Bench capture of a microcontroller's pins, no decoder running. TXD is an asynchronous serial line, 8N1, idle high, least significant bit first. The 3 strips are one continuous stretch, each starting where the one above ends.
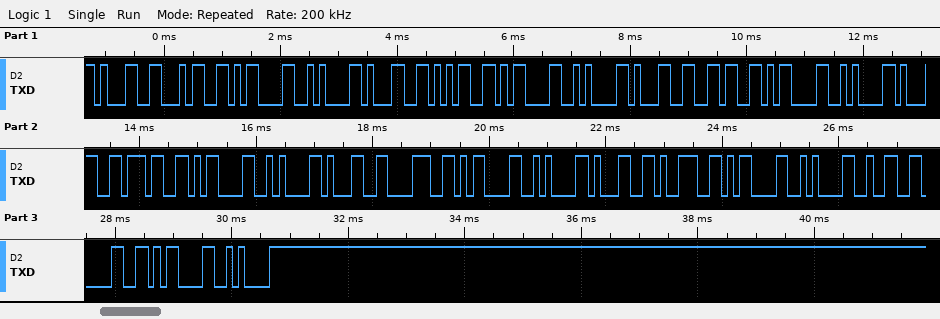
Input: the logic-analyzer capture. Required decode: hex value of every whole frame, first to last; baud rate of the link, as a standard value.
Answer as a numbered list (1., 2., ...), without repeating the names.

1. 31 34 0D 0A 31 35 0D 0A 31 36 0D 0A 31 37 0D 0A 31 38 0D 0A 31 39 0D 0A 32 30 0D 0A
2. 9600 baud
